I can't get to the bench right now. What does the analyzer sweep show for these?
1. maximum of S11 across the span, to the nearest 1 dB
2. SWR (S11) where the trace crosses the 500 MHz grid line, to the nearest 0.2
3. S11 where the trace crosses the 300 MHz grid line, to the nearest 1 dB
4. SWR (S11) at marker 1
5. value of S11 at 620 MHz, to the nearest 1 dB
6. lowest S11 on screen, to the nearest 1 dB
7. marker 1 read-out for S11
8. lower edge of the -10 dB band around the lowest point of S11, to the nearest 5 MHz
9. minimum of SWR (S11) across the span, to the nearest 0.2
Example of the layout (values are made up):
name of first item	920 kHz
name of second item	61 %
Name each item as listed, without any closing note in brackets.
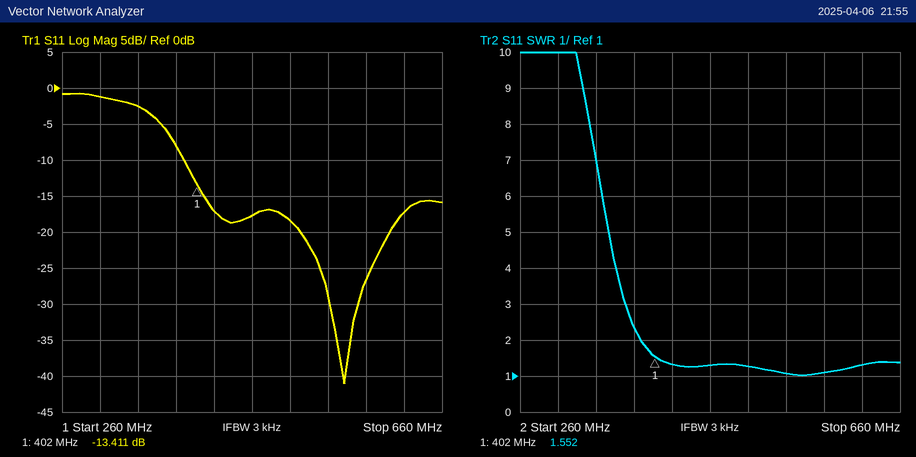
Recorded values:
maximum of S11 across the span, to the nearest 1 dB	-1 dB
SWR (S11) where the trace crosses the 500 MHz grid line, to the nearest 0.2	1.2
S11 where the trace crosses the 300 MHz grid line, to the nearest 1 dB	-1 dB
SWR (S11) at marker 1	1.552
value of S11 at 620 MHz, to the nearest 1 dB	-17 dB
lowest S11 on screen, to the nearest 1 dB	-41 dB
marker 1 read-out for S11	-13.411 dB
lower edge of the -10 dB band around the lowest point of S11, to the nearest 5 MHz	390 MHz
minimum of SWR (S11) across the span, to the nearest 0.2	1.0
